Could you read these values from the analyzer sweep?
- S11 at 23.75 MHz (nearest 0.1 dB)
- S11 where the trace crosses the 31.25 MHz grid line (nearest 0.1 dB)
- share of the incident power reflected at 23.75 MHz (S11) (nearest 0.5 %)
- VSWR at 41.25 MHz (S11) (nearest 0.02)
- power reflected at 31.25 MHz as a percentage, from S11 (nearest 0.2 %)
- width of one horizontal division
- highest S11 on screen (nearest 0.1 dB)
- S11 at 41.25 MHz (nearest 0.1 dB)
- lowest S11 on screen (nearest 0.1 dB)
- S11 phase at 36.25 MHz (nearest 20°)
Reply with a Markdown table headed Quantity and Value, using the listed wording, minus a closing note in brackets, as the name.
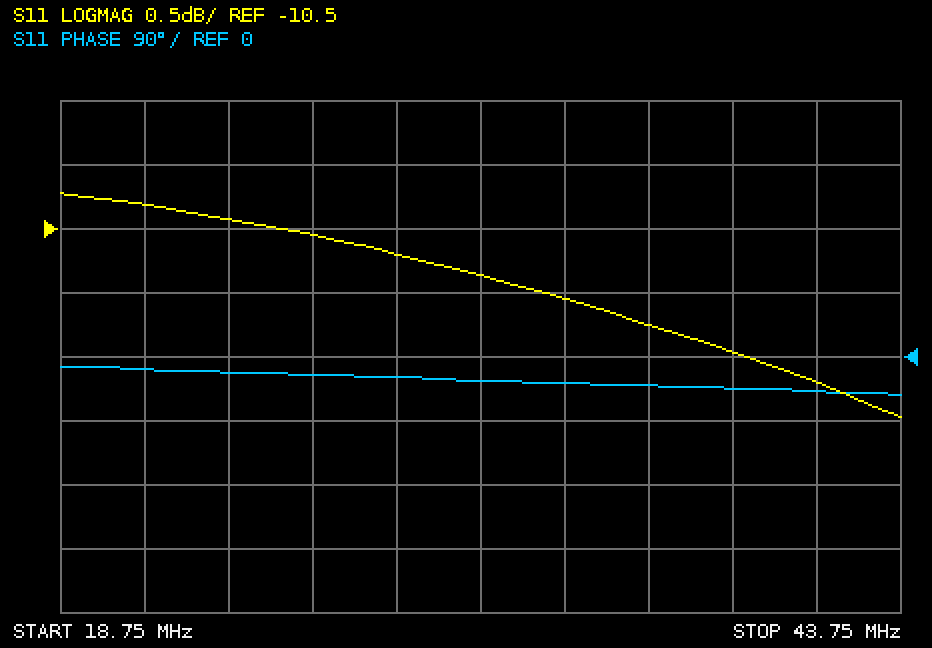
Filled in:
| Quantity | Value |
|---|---|
| S11 at 23.75 MHz | -10.4 dB |
| S11 where the trace crosses the 31.25 MHz grid line | -10.9 dB |
| share of the incident power reflected at 23.75 MHz (S11) | 9.0 % |
| VSWR at 41.25 MHz (S11) | 1.70 |
| power reflected at 31.25 MHz as a percentage, from S11 | 8.2 % |
| width of one horizontal division | 2.5 MHz |
| highest S11 on screen | -10.2 dB |
| S11 at 41.25 MHz | -11.7 dB |
| lowest S11 on screen | -12.0 dB |
| S11 phase at 36.25 MHz | -40° |
